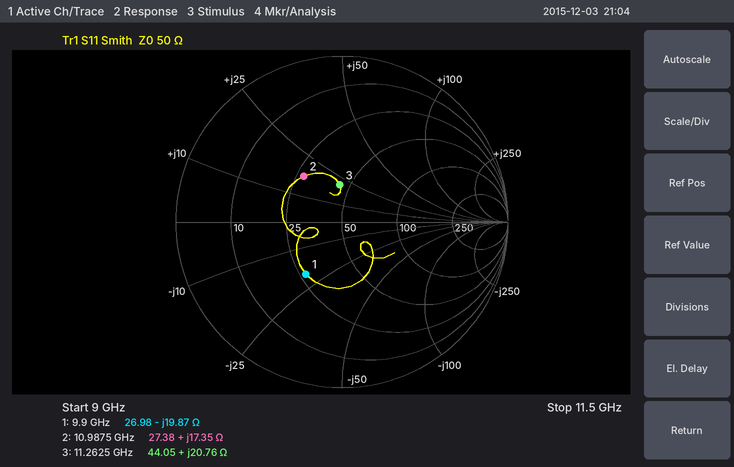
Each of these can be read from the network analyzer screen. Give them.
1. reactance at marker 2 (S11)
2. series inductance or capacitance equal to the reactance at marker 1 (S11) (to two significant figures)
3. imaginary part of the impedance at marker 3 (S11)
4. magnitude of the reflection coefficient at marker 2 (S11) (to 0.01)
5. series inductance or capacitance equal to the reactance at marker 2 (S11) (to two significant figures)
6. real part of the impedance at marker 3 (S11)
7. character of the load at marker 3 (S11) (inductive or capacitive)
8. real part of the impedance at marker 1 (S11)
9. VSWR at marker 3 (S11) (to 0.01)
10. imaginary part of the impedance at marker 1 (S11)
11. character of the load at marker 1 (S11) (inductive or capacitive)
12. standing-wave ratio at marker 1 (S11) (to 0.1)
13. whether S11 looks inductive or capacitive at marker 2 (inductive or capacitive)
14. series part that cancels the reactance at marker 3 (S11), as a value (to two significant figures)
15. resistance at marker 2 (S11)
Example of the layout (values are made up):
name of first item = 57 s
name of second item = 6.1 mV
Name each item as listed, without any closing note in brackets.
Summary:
reactance at marker 2 = +17.35 Ω
series inductance or capacitance equal to the reactance at marker 1 (S11) = 810 fF
imaginary part of the impedance at marker 3 = +20.76 Ω
magnitude of the reflection coefficient at marker 2 (S11) = 0.36
series inductance or capacitance equal to the reactance at marker 2 (S11) = 250 pH
real part of the impedance at marker 3 = 44.05 Ω
character of the load at marker 3 (S11) = inductive
real part of the impedance at marker 1 = 26.98 Ω
VSWR at marker 3 (S11) = 1.58
imaginary part of the impedance at marker 1 = -19.87 Ω
character of the load at marker 1 (S11) = capacitive
standing-wave ratio at marker 1 (S11) = 2.2
whether S11 looks inductive or capacitive at marker 2 = inductive
series part that cancels the reactance at marker 3 (S11), as a value = 680 fF
resistance at marker 2 = 27.38 Ω
